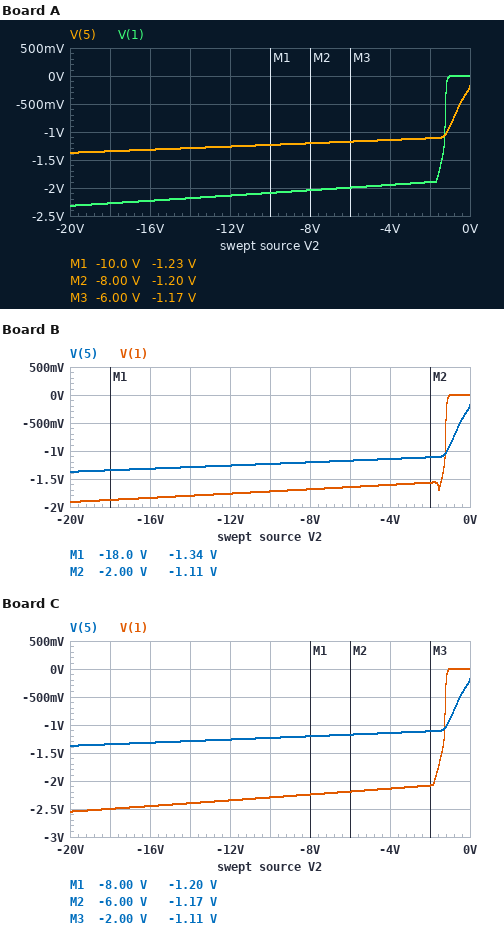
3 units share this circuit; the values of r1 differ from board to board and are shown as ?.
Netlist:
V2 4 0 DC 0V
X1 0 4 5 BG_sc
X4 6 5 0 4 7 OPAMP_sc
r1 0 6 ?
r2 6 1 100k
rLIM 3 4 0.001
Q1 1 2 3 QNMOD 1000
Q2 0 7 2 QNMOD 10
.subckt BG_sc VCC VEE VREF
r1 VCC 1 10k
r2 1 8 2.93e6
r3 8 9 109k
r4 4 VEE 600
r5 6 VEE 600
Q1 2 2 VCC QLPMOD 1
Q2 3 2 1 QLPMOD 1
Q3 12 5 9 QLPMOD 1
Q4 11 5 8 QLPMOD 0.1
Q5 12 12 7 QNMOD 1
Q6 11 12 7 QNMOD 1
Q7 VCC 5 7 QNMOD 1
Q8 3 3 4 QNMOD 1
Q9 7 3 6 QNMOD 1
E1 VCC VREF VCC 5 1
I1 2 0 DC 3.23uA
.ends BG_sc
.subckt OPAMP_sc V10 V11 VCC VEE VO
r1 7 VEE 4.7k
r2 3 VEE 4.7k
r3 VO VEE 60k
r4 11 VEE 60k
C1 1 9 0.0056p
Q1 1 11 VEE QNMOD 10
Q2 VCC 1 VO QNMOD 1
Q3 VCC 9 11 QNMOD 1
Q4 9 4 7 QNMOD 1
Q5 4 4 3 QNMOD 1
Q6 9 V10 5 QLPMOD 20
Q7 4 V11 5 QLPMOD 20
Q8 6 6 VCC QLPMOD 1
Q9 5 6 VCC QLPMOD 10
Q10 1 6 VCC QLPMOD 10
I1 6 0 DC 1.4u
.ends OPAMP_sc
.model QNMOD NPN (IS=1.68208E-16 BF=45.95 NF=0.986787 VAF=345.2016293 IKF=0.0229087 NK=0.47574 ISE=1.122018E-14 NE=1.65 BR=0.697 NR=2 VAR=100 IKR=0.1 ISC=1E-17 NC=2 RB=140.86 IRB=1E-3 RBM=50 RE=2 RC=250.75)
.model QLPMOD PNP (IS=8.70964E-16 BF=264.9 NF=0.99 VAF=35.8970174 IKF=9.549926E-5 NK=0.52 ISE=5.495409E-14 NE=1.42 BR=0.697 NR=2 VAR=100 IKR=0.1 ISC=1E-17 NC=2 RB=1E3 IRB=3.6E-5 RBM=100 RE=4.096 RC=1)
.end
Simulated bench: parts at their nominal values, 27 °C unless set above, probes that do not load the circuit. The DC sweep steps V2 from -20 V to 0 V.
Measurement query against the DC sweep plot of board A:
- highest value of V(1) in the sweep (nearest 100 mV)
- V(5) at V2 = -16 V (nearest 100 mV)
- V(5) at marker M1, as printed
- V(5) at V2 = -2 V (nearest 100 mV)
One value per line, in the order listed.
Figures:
0 V
-1.3 V
-1.23 V
-1.1 V
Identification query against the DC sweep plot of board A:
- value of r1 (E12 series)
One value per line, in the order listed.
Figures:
150 kΩ
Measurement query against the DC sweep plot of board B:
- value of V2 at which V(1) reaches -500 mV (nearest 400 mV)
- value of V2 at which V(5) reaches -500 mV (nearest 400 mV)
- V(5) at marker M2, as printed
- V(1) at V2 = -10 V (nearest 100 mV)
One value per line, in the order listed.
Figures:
-1.2 V
-400 mV
-1.11 V
-1.7 V
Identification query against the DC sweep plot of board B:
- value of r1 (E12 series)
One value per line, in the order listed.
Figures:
270 kΩ
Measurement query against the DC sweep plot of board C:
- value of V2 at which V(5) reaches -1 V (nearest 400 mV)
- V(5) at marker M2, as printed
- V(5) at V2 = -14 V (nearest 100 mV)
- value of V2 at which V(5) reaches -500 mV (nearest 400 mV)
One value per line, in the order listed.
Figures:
-1.2 V
-1.17 V
-1.3 V
-400 mV
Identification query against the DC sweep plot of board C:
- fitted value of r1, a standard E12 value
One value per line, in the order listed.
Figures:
120 kΩ
